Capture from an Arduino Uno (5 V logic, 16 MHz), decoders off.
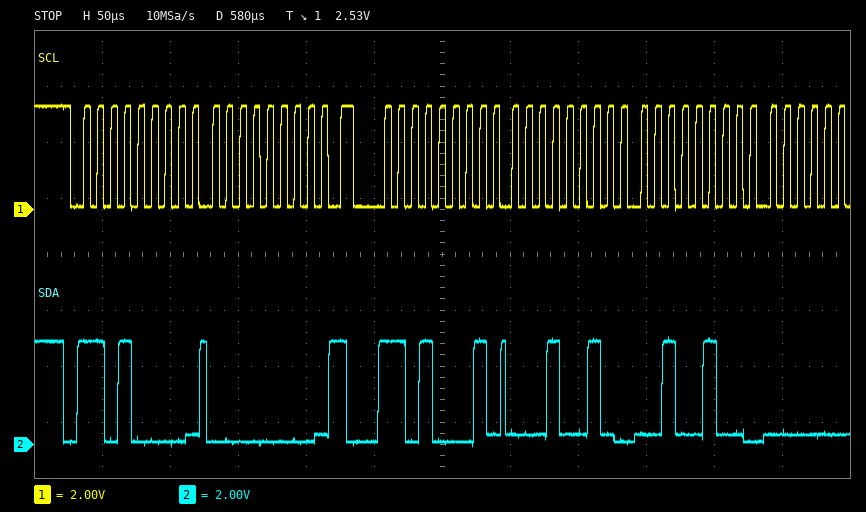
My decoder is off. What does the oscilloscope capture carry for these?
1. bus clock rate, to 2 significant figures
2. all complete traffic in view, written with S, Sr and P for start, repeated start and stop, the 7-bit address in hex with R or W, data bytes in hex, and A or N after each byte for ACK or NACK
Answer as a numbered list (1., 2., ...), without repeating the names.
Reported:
1. 100 kHz
2. S 68W A 00 A Sr 68R A 12 A 24 A
